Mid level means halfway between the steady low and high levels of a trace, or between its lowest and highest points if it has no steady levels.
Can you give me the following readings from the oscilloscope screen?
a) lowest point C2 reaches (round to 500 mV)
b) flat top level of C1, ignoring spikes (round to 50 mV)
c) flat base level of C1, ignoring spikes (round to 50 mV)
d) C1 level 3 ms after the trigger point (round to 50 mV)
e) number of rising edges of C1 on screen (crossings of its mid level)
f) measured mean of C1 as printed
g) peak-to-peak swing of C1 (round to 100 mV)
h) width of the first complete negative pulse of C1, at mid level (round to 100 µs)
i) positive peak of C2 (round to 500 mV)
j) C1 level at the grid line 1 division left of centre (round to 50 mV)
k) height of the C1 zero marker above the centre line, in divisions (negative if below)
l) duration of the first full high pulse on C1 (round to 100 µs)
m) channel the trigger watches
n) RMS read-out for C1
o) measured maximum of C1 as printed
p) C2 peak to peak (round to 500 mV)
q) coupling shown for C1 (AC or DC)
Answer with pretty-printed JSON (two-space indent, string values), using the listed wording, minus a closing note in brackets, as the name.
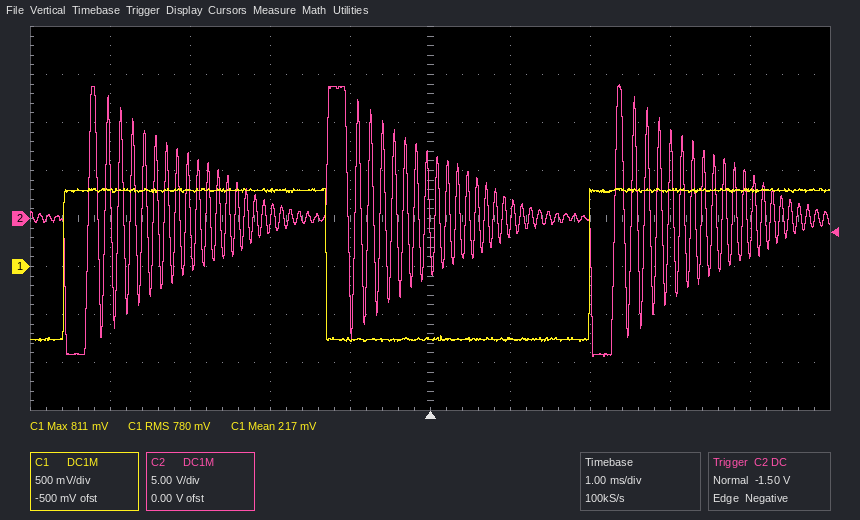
{
  "lowest point C2 reaches": "-14.5 V",
  "flat top level of C1, ignoring spikes": "800 mV",
  "flat base level of C1, ignoring spikes": "-750 mV",
  "C1 level 3 ms after the trigger point": "800 mV",
  "number of rising edges of C1 on screen": "2",
  "measured mean of C1 as printed": "217 mV",
  "peak-to-peak swing of C1": "1.60 V",
  "width of the first complete negative pulse of C1, at mid level": "3.3 ms",
  "positive peak of C2": "14.0 V",
  "C1 level at the grid line 1 division left of centre": "-750 mV",
  "height of the C1 zero marker above the centre line, in divisions": "-1.0 div",
  "duration of the first full high pulse on C1": "3.3 ms",
  "channel the trigger watches": "C2",
  "RMS read-out for C1": "780 mV",
  "measured maximum of C1 as printed": "811 mV",
  "C2 peak to peak": "28.5 V",
  "coupling shown for C1": "DC"
}
